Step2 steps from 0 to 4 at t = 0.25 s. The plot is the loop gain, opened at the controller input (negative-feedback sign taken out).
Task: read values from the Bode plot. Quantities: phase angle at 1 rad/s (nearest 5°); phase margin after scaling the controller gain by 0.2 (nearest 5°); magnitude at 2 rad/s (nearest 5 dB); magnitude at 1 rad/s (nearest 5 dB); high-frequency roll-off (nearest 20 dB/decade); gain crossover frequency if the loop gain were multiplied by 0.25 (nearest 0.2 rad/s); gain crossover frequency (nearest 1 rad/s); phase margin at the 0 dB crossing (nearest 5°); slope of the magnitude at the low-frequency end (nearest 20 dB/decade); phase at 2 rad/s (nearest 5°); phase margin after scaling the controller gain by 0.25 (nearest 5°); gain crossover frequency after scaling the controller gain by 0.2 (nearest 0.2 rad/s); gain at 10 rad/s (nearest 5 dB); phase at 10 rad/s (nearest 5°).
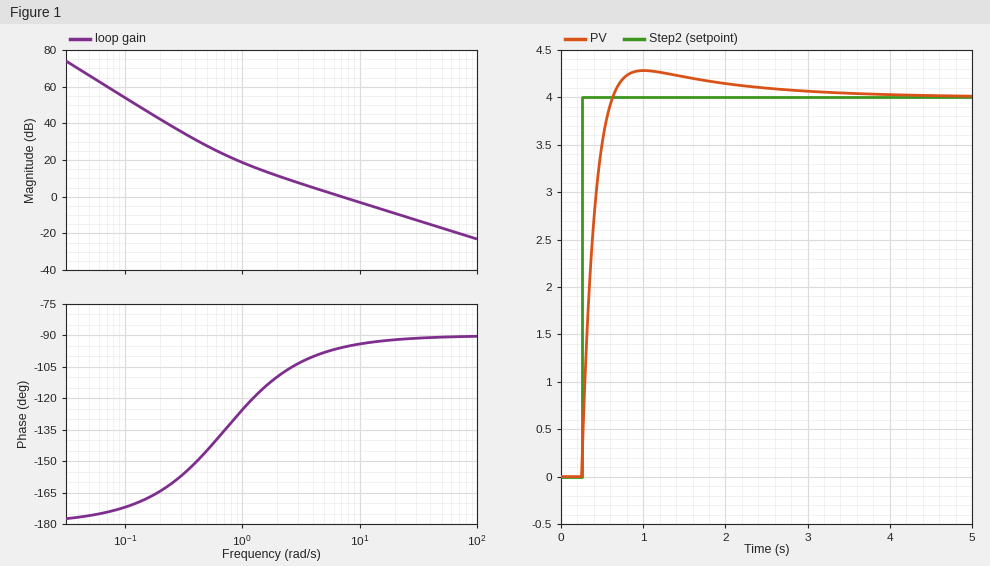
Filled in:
-125°
65°
10 dB
20 dB
-20 dB/decade
1.8 rad/s
7 rad/s
85°
-40 dB/decade
-110°
70°
1.6 rad/s
-5 dB
-95°
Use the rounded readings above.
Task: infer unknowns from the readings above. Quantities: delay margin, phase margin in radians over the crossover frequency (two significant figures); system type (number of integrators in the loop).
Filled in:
0.21 s
2
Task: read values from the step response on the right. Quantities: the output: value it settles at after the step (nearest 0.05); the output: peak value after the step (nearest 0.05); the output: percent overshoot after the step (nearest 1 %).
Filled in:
4.00
4.30
7 %
